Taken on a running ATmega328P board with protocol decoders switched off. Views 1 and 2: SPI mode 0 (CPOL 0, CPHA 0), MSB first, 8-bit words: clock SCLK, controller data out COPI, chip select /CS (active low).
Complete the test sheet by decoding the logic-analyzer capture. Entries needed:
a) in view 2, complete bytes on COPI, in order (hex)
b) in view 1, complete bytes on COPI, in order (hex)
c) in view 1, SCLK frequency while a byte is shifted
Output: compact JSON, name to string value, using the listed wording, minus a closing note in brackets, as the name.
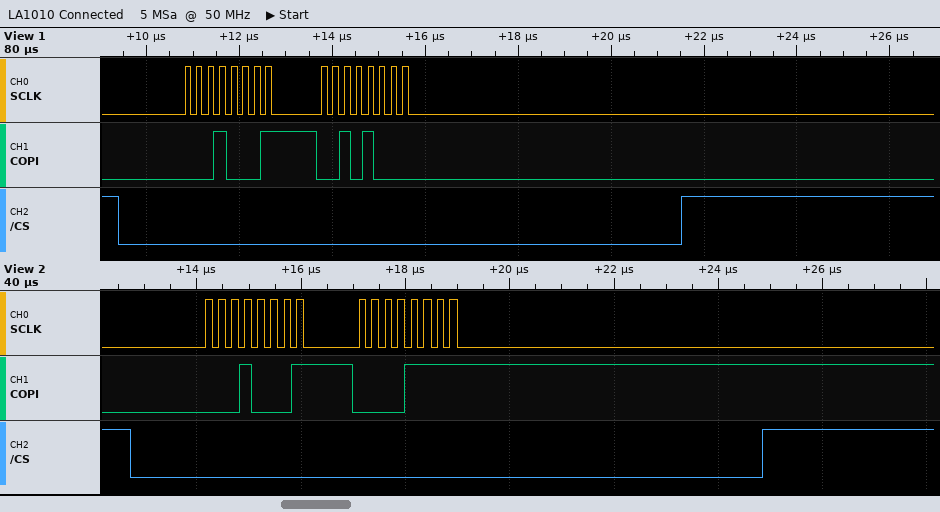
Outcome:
{"in view 2, complete bytes on COPI, in order": "0x11 0x0F", "in view 1, complete bytes on COPI, in order": "11 28", "in view 1, SCLK frequency while a byte is shifted": "4 MHz"}
